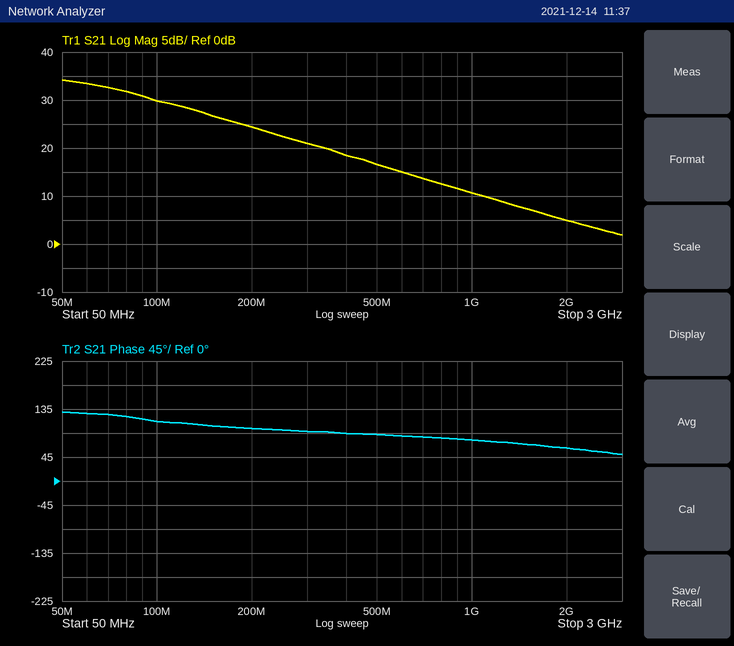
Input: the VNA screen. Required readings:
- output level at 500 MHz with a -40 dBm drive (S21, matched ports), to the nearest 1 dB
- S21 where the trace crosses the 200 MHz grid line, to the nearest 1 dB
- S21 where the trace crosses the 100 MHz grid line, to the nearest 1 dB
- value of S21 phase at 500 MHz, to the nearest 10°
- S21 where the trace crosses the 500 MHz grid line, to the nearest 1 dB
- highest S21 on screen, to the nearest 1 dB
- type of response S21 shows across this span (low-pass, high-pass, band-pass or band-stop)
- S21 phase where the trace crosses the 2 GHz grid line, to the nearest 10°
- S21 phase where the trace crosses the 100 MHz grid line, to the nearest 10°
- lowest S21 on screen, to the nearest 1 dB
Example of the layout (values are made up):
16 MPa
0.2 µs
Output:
-23 dBm
24 dB
30 dB
90°
17 dB
34 dB
low-pass
60°
110°
2 dB
